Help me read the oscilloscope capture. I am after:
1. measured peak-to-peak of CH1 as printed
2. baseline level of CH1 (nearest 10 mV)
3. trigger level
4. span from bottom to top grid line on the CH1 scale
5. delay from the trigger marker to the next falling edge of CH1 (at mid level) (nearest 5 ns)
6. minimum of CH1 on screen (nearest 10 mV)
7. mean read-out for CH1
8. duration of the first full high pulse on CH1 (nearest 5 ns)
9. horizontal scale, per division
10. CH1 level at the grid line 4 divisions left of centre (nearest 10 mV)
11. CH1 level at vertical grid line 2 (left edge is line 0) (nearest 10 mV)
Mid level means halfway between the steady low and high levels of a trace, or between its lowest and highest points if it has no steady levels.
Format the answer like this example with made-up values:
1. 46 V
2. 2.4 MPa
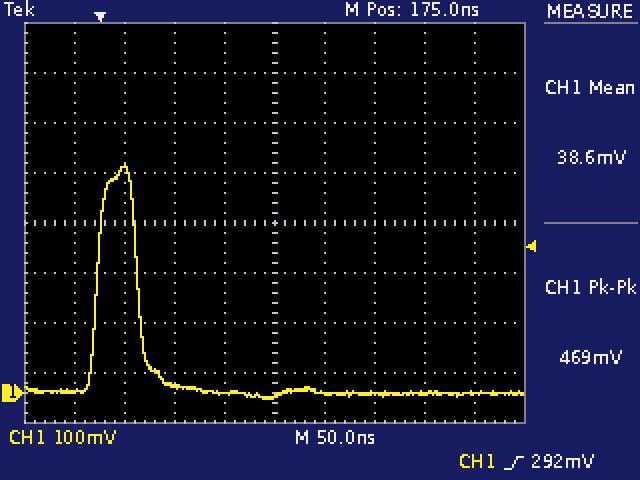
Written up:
1. 469 mV
2. 0 mV
3. 292 mV
4. 800 mV
5. 40 ns
6. -10 mV
7. 38.6 mV
8. 40 ns
9. 50 ns
10. 0 mV
11. 450 mV
